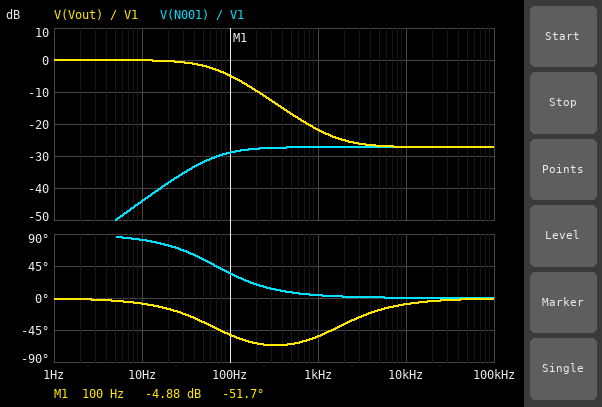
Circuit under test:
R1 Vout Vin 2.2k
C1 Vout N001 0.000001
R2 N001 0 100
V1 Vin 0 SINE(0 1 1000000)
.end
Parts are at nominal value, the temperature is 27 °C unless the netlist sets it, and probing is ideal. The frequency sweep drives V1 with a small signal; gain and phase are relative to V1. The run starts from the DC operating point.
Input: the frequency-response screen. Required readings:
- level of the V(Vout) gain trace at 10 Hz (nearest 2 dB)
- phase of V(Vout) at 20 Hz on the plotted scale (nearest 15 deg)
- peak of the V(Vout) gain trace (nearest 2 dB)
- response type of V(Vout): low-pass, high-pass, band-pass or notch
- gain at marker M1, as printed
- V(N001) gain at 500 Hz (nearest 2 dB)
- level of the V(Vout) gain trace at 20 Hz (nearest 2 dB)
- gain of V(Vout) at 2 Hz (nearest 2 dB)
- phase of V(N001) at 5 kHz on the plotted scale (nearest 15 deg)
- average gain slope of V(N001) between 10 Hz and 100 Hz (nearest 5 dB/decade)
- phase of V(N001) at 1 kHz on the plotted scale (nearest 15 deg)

0 dB
-15 deg
0 dB
low-pass
-4.88 dB
-28 dB
0 dB
0 dB
0 deg
15 dB/decade
0 deg
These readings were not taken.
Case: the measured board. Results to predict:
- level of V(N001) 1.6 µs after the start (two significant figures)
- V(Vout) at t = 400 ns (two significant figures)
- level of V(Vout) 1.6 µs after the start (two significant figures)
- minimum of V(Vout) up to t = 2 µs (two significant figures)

-26 mV
26 mV
-25 mV
-43 mV
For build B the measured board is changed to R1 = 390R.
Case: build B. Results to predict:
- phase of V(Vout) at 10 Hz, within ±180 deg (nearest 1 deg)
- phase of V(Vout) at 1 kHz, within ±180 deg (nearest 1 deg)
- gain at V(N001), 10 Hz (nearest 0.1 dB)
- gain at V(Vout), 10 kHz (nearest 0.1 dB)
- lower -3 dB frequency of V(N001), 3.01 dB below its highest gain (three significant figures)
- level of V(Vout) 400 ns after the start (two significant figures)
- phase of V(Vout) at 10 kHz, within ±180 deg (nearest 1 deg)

-1 deg
-40 deg
-44.0 dB
-13.7 dB
325 Hz
120 mV
-7 deg
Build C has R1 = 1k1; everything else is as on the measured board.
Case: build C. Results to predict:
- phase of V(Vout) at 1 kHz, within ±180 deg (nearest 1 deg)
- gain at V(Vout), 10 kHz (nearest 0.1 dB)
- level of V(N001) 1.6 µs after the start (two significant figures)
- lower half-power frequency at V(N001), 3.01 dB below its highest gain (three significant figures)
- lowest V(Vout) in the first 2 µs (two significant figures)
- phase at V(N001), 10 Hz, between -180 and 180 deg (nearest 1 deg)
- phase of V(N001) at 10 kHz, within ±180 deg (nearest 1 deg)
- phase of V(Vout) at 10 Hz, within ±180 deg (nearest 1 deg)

-50 deg
-21.5 dB
-49 mV
133 Hz
-83 mV
86 deg
1 deg
-4 deg
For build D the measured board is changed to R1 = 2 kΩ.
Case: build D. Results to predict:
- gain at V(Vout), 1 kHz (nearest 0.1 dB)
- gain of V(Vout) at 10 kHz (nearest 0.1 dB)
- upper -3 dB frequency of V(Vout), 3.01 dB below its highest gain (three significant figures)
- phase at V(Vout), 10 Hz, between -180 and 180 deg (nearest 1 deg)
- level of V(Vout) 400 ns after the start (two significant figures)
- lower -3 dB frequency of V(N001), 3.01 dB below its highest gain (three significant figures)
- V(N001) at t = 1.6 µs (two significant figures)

-21.0 dB
-26.3 dB
76.0 Hz
-7 deg
28 mV
75.8 Hz
-28 mV
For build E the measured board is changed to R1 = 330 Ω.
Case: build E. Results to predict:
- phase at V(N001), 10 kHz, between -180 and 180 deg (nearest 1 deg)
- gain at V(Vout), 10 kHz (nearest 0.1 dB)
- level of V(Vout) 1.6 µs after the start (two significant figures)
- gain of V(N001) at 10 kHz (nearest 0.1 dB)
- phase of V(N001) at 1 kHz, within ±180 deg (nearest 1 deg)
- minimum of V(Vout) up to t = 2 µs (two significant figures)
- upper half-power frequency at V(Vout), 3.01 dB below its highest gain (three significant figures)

2 deg
-12.6 dB
-140 mV
-12.7 dB
20 deg
-230 mV
392 Hz
